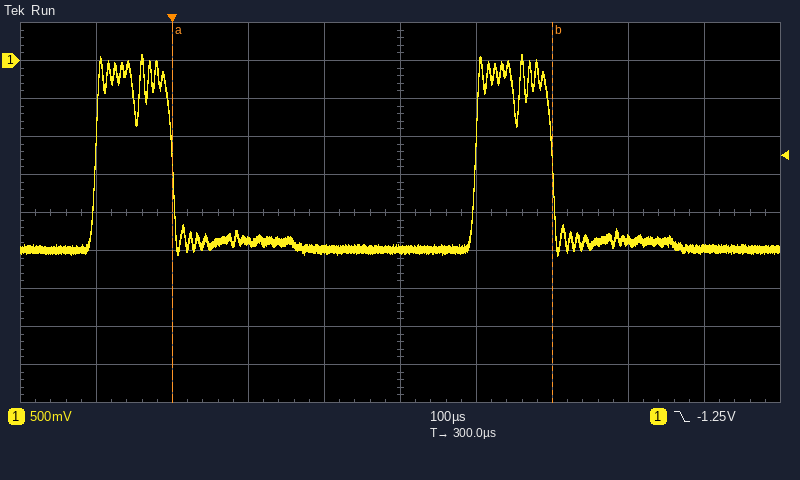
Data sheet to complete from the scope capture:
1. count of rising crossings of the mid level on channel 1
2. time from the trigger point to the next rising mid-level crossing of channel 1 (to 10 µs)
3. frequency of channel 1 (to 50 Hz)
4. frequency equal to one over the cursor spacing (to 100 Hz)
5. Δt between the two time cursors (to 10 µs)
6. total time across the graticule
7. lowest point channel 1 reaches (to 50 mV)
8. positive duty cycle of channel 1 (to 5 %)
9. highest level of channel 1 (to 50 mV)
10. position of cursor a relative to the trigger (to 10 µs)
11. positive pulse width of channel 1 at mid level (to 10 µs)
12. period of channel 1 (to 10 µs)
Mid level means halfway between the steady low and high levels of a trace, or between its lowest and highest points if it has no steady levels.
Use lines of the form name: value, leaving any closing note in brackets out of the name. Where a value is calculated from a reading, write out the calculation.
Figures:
count of rising crossings of the mid level on channel 1: 2
time from the trigger point to the next rising mid-level crossing of channel 1: 400 µs
frequency of channel 1: 1 / 500 µs ≈ 2.00 kHz
frequency equal to one over the cursor spacing: 1 / 500 µs ≈ 2.0 kHz
Δt between the two time cursors: 500 µs
total time across the graticule: 1 ms
lowest point channel 1 reaches: -2.60 V
positive duty cycle of channel 1: 100 µs / 500 µs ≈ 20 %
highest level of channel 1: 100 mV
position of cursor a relative to the trigger: 0 µs
positive pulse width of channel 1 at mid level: 100 µs
period of channel 1: 500 µs
